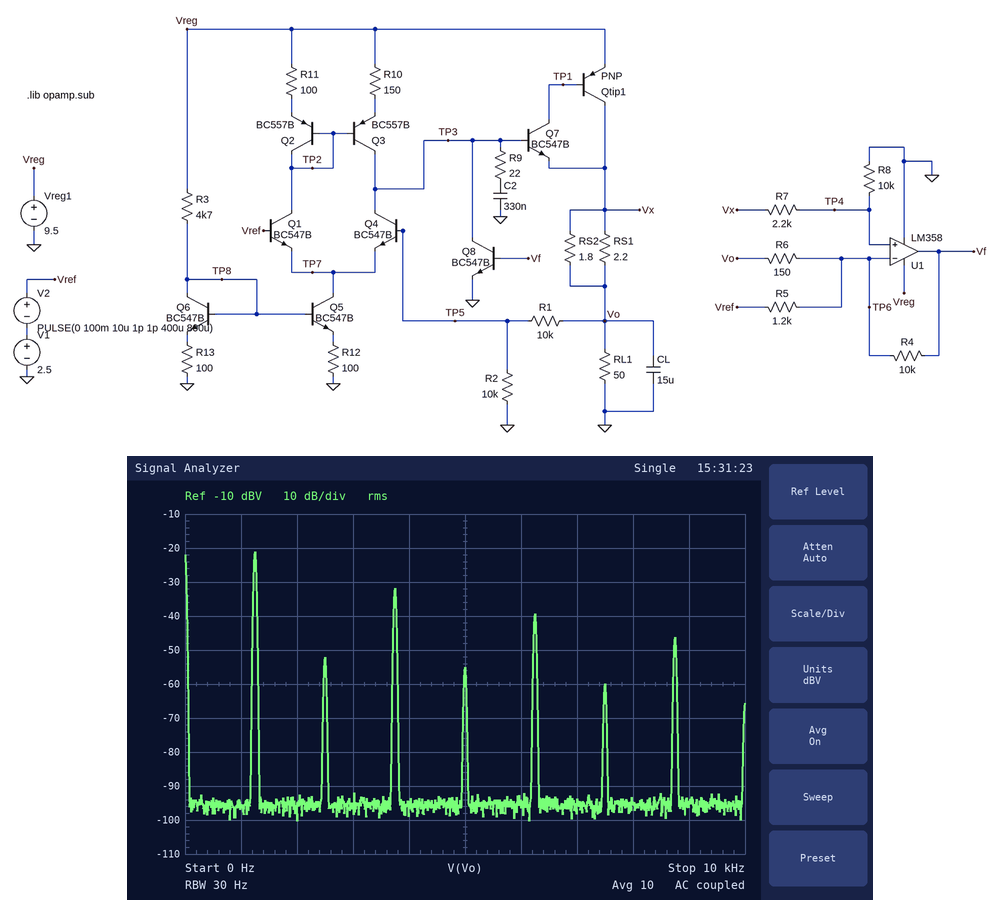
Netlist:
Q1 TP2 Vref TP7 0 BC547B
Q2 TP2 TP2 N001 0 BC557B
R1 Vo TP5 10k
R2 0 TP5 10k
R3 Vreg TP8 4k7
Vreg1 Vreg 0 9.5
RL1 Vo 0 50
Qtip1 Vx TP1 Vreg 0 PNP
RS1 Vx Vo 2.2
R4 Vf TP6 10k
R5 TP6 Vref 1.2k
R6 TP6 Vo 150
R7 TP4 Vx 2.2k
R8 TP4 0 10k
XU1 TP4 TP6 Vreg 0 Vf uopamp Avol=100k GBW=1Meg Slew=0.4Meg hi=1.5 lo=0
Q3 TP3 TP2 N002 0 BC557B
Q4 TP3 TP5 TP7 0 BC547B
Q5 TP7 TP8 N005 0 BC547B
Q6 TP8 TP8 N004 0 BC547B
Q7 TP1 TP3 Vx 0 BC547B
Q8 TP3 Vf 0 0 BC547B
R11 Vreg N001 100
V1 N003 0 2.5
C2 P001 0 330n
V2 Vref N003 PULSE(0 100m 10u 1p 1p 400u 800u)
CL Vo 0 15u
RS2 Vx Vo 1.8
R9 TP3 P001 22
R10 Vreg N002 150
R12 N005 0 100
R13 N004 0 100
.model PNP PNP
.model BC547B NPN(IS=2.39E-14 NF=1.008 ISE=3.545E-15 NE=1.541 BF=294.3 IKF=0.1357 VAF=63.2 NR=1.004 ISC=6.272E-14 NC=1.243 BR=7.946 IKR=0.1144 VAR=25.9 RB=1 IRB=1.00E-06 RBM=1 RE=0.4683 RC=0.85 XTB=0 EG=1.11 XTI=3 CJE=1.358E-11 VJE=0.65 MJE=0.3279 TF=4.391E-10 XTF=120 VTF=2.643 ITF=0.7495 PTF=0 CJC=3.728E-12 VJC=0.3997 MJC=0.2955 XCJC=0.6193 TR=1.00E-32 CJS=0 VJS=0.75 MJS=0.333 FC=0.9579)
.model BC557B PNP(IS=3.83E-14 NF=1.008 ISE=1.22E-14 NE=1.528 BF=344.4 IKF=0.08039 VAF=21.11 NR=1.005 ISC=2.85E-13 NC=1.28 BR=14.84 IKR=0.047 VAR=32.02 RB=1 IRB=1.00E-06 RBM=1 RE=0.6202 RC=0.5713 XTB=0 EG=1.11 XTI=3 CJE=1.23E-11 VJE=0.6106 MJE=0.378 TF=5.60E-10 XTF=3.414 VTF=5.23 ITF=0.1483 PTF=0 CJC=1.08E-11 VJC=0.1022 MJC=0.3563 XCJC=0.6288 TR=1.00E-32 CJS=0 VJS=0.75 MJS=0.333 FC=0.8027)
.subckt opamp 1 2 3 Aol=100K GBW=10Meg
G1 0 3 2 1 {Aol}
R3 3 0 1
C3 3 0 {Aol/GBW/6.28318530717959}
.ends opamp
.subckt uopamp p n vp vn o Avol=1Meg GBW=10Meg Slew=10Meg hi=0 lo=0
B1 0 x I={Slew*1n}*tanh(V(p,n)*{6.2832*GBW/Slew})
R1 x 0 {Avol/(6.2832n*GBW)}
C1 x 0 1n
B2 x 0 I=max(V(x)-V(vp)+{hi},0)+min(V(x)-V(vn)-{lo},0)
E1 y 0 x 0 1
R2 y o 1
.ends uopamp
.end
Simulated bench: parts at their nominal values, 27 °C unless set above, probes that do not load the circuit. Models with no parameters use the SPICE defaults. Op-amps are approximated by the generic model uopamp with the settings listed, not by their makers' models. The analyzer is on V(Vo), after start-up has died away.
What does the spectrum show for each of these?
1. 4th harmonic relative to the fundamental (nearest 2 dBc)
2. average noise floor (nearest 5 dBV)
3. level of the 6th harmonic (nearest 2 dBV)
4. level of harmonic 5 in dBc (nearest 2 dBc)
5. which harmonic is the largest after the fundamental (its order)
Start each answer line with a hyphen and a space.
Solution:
- -34 dBc
- -95 dBV
- -60 dBV
- -18 dBc
- 3
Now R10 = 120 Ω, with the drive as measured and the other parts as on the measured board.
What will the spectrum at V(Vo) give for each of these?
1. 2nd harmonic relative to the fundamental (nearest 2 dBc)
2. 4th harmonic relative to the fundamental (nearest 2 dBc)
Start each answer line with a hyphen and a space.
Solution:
- -40 dBc
- -42 dBc
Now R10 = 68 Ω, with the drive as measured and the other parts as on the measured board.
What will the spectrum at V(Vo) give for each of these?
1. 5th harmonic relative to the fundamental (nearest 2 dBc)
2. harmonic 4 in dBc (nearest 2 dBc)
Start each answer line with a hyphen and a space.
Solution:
- -16 dBc
- -32 dBc
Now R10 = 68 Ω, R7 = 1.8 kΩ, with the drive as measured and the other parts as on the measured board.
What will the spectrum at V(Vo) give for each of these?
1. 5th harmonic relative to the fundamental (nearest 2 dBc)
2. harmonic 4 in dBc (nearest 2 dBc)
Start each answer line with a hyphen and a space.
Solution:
- -16 dBc
- -32 dBc
